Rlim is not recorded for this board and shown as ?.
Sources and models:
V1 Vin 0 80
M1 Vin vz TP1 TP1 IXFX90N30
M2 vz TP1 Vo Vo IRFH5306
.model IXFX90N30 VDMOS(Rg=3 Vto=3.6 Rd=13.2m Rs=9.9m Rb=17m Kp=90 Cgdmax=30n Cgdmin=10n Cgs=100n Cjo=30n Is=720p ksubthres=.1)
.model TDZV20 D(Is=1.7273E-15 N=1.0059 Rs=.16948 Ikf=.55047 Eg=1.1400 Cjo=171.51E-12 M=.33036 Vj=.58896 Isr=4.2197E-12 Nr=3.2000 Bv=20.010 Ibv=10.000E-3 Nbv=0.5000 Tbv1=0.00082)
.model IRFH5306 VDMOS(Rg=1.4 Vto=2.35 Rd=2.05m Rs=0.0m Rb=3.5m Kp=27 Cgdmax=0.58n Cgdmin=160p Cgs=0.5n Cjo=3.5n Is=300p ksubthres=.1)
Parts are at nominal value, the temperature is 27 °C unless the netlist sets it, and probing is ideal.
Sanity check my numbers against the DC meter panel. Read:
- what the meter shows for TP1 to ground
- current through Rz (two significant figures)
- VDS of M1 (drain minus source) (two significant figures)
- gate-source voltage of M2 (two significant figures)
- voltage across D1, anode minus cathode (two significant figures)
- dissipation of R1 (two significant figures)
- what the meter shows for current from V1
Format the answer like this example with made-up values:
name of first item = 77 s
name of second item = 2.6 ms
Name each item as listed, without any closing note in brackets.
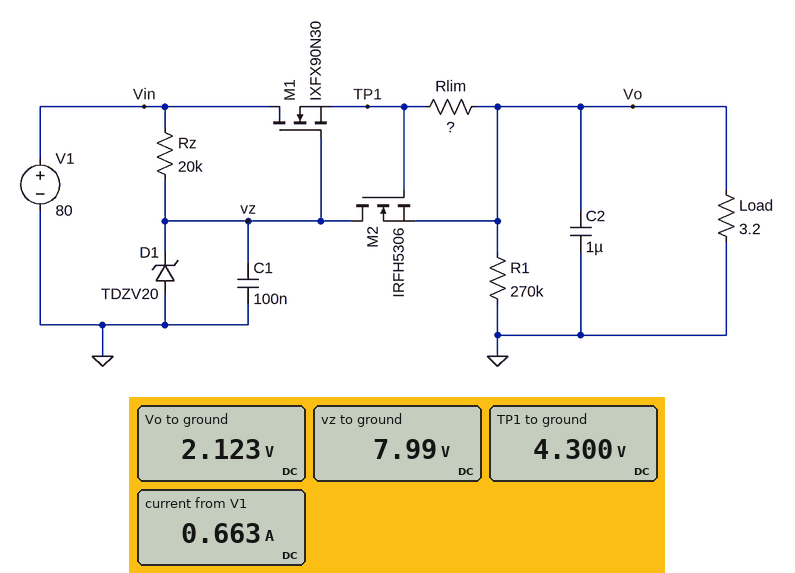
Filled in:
what the meter shows for TP1 to ground = 4.300 V
current through Rz = 3.6 mA
VDS of M1 (drain minus source) = 76 V
gate-source voltage of M2 = 2.2 V
voltage across D1, anode minus cathode = -8.0 V
dissipation of R1 = 17 µW
what the meter shows for current from V1 = 0.663 A
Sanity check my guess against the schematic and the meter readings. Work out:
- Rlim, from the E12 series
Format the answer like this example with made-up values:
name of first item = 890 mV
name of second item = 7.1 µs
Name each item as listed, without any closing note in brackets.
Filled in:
Rlim, from the E12 series = 3.3 Ω
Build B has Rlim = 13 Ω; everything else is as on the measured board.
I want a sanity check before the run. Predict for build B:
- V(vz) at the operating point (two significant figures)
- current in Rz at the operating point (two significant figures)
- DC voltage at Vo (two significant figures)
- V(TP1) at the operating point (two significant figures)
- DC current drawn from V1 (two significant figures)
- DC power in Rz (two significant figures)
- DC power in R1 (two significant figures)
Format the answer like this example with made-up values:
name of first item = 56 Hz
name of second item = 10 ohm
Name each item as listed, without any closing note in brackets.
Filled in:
V(vz) at the operating point = 6.3 V
current in Rz at the operating point = 3.7 mA
DC voltage at Vo = 550 mV
V(TP1) at the operating point = 2.7 V
DC current drawn from V1 = 170 mA
DC power in Rz = 270 mW
DC power in R1 = 1.1 µW
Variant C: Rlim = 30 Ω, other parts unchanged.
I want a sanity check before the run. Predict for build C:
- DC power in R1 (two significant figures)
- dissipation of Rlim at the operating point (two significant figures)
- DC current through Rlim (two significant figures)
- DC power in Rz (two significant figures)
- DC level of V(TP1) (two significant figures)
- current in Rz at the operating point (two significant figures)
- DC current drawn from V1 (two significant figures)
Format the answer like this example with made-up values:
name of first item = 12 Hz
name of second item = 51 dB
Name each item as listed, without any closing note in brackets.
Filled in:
DC power in R1 = 220 nW
dissipation of Rlim at the operating point = 160 mW
DC current through Rlim = 73 mA
DC power in Rz = 270 mW
DC level of V(TP1) = 2.4 V
current in Rz at the operating point = 3.7 mA
DC current drawn from V1 = 76 mA
